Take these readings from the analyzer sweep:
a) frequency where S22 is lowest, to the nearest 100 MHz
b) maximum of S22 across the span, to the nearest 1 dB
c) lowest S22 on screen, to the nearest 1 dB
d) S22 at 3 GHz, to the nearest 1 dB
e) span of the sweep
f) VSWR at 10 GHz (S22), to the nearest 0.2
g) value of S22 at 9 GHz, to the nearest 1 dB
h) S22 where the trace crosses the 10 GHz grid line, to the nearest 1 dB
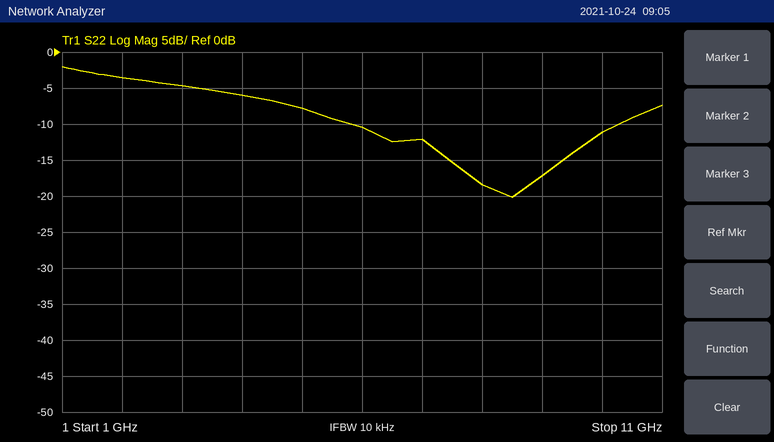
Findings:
8.5 GHz
-2 dB
-20 dB
-5 dB
10 GHz
1.8
-17 dB
-11 dB
